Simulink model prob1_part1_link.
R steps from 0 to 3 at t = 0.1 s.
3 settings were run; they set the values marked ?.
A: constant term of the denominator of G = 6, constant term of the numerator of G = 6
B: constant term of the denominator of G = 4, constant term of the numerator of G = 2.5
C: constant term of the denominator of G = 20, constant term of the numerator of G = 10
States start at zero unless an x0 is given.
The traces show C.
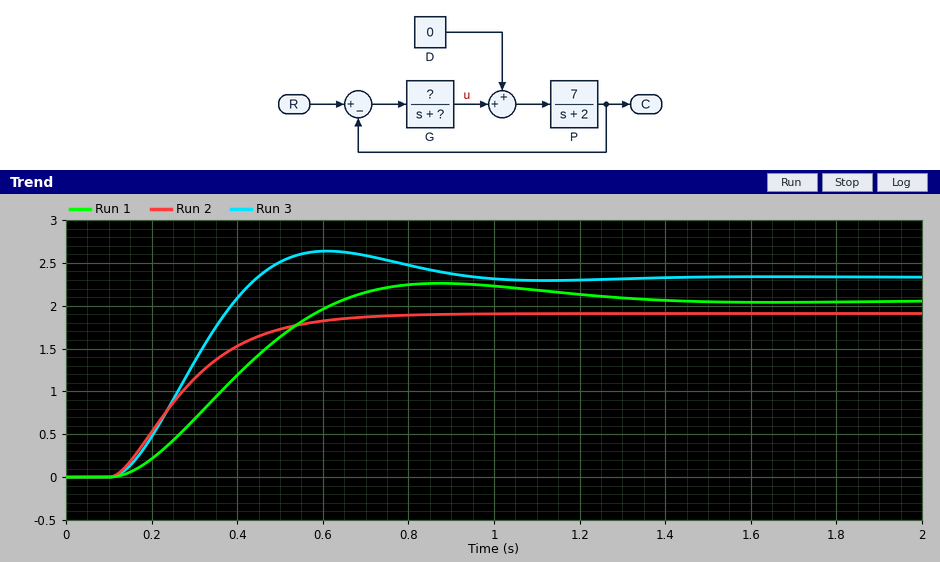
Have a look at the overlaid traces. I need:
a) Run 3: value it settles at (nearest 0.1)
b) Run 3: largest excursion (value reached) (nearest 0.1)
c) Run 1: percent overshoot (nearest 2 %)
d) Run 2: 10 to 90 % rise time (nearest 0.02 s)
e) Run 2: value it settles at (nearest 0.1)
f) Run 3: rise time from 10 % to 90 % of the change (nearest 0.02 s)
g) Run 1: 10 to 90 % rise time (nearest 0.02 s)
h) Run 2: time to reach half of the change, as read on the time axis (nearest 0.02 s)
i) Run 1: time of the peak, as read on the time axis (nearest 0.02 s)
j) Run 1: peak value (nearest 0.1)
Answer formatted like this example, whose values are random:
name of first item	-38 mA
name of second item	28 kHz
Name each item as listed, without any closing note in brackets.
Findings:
Run 3: value it settles at	2.3
Run 3: largest excursion (value reached)	2.6
Run 1: percent overshoot	10 %
Run 2: 10 to 90 % rise time	0.34 s
Run 2: value it settles at	1.9
Run 3: rise time from 10 % to 90 % of the change	0.24 s
Run 1: 10 to 90 % rise time	0.36 s
Run 2: time to reach half of the change, as read on the time axis	0.26 s
Run 1: time of the peak, as read on the time axis	0.88 s
Run 1: peak value	2.3
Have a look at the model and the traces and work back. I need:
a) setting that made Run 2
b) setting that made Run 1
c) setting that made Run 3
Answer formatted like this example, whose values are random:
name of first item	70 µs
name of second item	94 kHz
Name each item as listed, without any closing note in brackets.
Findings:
setting that made Run 2	C
setting that made Run 1	B
setting that made Run 3	A
